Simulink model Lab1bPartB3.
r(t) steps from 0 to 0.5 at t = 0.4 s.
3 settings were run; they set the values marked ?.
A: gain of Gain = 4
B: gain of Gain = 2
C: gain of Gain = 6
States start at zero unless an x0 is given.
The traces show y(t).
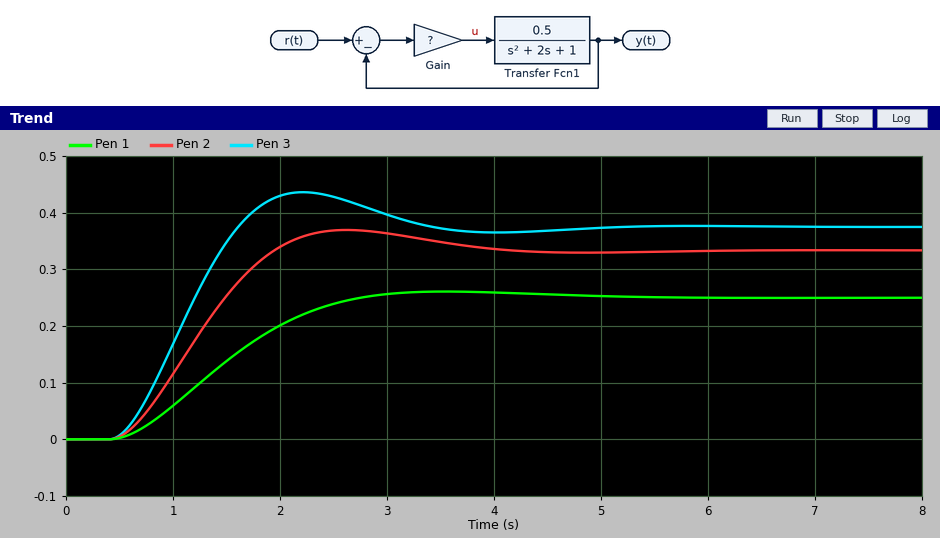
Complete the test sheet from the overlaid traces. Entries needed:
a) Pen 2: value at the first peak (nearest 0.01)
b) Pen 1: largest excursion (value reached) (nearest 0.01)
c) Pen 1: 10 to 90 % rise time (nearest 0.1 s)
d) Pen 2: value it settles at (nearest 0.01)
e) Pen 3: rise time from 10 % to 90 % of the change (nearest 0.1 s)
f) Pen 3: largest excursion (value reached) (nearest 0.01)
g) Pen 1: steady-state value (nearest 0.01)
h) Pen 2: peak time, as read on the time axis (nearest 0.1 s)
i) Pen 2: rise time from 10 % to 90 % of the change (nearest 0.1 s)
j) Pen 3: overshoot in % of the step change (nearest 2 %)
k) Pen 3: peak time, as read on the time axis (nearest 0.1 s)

0.37
0.26
1.5 s
0.33
0.8 s
0.44
0.25
2.6 s
1.0 s
16 %
2.2 s
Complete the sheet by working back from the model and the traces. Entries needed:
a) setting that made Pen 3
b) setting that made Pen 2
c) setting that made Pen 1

C
A
B
